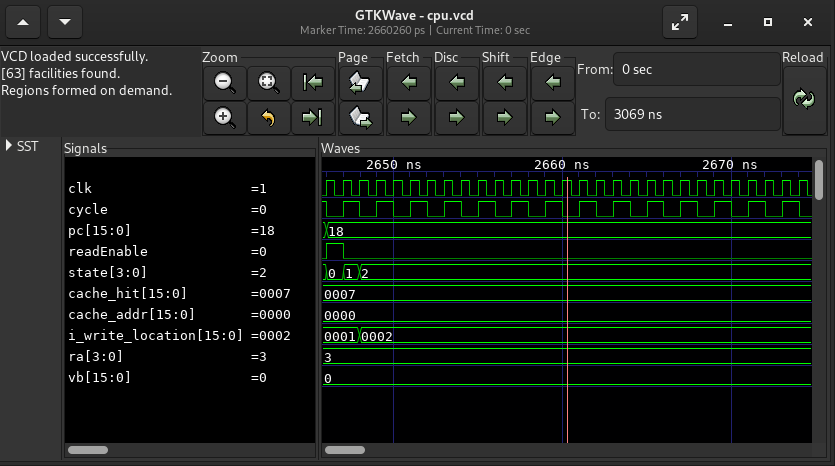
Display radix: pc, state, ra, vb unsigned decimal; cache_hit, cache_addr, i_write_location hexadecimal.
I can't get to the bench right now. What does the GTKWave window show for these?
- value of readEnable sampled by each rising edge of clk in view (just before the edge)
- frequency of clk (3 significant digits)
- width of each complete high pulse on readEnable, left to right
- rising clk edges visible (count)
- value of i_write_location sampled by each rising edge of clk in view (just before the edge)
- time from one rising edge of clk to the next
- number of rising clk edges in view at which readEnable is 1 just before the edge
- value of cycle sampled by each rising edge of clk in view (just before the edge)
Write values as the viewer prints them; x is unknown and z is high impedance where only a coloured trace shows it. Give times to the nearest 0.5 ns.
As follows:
0 1 0 0 0 0 0 0 0 0 0 0 0 0 0 0 0 0 0 0 0 0 0 0 0 0 0 0 0
1.00 GHz
1 ns
29
0001, 0001, 0001, 0002, 0002, 0002, 0002, 0002, 0002, 0002, 0002, 0002, 0002, 0002, 0002, 0002, 0002, 0002, 0002, 0002, 0002, 0002, 0002, 0002, 0002, 0002, 0002, 0002, 0002
1 ns
1
1 0 1 0 1 0 1 0 1 0 1 0 1 0 1 0 1 0 1 0 1 0 1 0 1 0 1 0 1
